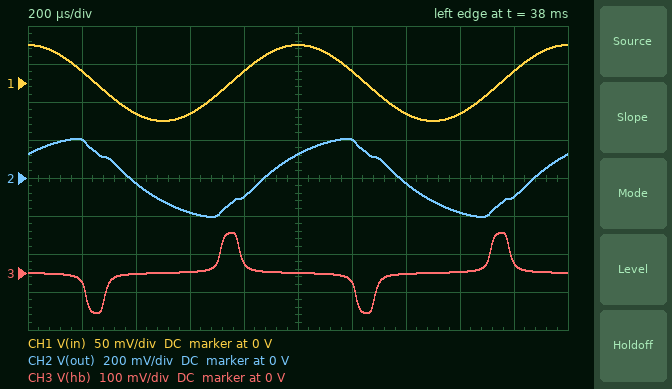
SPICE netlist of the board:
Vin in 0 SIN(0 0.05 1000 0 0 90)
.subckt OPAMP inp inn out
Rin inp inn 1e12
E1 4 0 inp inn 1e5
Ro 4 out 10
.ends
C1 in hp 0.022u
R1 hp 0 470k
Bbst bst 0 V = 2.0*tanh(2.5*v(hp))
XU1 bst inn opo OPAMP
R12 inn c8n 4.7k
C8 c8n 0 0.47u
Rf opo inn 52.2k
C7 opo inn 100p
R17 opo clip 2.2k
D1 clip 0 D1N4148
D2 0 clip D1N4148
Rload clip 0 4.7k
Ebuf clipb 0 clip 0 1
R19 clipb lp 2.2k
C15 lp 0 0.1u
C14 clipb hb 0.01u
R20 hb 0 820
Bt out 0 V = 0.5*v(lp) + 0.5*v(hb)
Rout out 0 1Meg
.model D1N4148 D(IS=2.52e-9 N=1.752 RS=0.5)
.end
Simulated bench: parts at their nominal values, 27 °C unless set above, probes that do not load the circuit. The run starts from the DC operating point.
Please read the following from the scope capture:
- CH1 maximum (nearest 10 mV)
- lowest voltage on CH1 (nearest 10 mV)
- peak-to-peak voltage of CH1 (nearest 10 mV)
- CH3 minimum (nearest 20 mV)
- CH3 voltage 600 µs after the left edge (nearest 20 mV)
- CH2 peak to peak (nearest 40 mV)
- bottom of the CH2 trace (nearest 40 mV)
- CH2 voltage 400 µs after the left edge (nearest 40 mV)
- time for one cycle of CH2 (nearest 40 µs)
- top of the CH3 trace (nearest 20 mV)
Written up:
50 mV
-50 mV
100 mV
-100 mV
0 V
400 mV
-200 mV
-40 mV
1.00 ms
100 mV
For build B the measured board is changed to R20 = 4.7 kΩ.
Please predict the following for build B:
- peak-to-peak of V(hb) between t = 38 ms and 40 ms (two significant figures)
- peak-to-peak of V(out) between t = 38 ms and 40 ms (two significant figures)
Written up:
910 mV
390 mV
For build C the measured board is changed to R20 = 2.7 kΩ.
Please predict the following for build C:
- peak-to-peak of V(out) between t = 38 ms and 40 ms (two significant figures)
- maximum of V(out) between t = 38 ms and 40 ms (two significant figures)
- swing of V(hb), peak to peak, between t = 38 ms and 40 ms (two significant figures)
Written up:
400 mV
200 mV
620 mV
